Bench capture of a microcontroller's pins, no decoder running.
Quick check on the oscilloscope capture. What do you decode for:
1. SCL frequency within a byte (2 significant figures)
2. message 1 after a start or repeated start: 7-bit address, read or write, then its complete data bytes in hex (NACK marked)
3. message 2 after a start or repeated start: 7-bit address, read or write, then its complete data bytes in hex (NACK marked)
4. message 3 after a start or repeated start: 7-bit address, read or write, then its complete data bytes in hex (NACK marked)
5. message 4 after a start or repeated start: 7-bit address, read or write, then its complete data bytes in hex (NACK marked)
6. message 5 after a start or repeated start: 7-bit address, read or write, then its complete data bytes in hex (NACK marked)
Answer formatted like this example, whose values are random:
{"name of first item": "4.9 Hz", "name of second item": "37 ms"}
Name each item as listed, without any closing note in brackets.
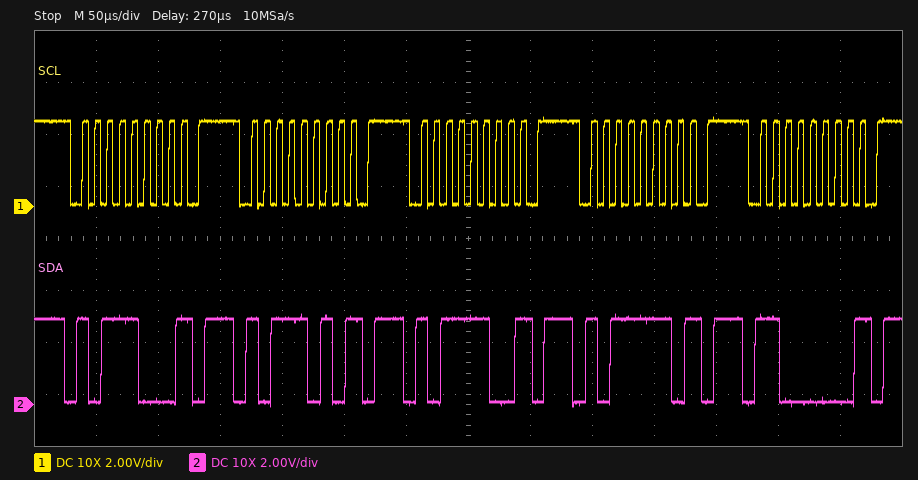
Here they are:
{"SCL frequency within a byte": "100 kHz", "message 1 after a start or repeated start: 7-bit address, read or write, then its complete data bytes in hex": "0x5C write NACK", "message 2 after a start or repeated start: 7-bit address, read or write, then its complete data bytes in hex": "0x5D write NACK", "message 3 after a start or repeated start: 7-bit address, read or write, then its complete data bytes in hex": "0x5E write NACK", "message 4 after a start or repeated start: 7-bit address, read or write, then its complete data bytes in hex": "0x5F write NACK", "message 5 after a start or repeated start: 7-bit address, read or write, then its complete data bytes in hex": "0x60 write NACK"}
